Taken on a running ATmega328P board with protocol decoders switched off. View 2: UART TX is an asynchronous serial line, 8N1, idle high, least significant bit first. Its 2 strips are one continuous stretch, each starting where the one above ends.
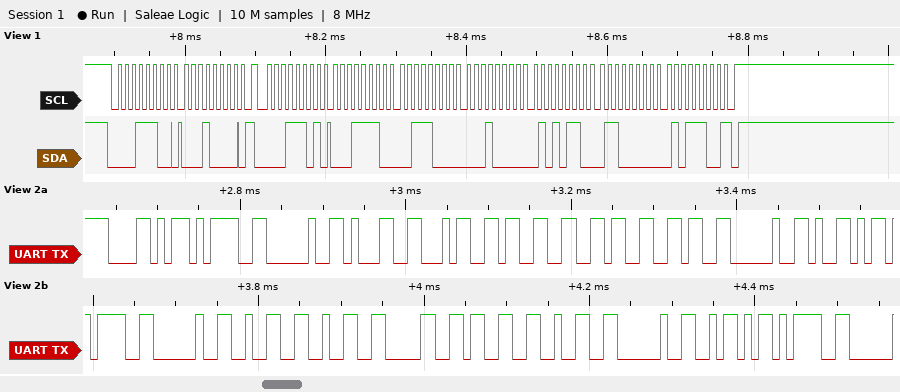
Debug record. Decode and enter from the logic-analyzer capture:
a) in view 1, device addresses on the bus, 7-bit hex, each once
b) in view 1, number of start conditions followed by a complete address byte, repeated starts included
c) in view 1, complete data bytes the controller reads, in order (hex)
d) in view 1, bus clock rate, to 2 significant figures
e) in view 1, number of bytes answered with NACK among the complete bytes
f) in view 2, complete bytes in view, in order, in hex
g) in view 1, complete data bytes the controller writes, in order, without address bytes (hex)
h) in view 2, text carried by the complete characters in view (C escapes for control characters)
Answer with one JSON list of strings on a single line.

["0x0E", "2", "1E 38 10 56 60 5C", "100 kHz", "1", "58 3D 20 31 34 33 36 36 20 59 3D 20 32 32 30 33 32 20 5A 3D", "10", "\"X= 14366 Y= 22032 Z=\""]
